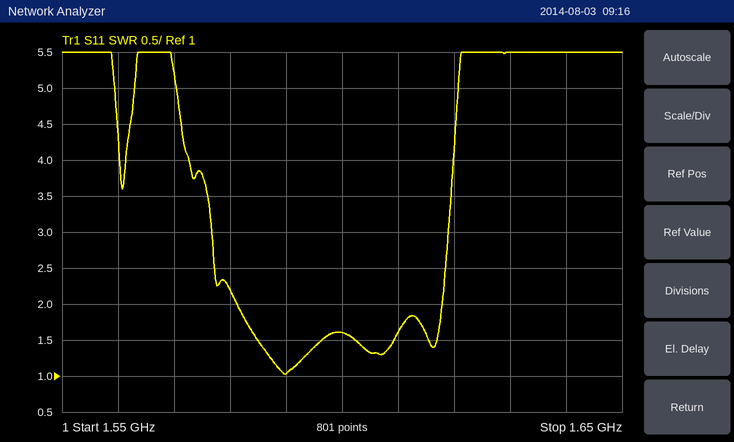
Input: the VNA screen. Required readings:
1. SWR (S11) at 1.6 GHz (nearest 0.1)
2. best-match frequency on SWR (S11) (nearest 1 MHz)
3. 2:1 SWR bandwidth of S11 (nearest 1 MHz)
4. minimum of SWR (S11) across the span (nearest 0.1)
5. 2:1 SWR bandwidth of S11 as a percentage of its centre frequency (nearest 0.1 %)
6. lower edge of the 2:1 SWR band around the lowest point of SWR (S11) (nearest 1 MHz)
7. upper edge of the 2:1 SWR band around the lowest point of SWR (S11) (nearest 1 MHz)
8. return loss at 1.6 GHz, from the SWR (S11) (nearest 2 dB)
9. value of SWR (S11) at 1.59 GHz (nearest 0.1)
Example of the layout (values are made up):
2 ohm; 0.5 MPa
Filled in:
1.6; 1.590 GHz; 37 MHz; 1.0; 2.3 %; 1.581 GHz; 1.618 GHz; 12 dB; 1.0
